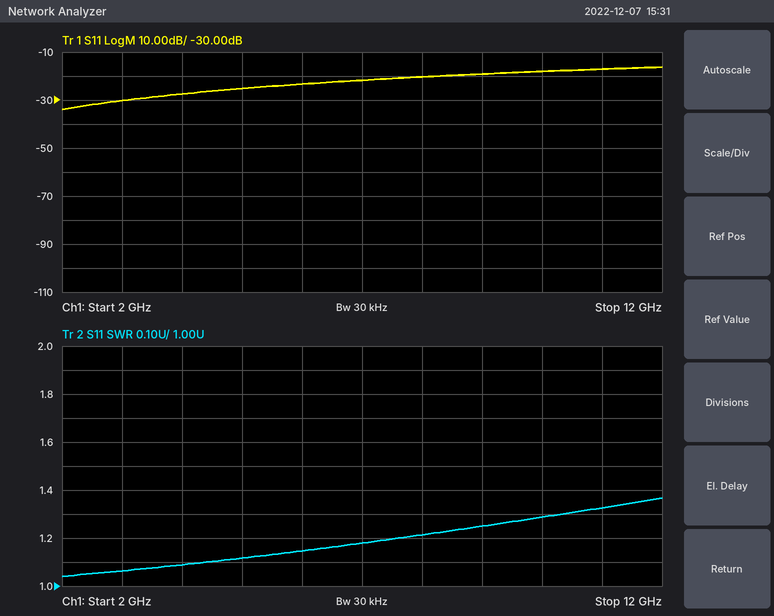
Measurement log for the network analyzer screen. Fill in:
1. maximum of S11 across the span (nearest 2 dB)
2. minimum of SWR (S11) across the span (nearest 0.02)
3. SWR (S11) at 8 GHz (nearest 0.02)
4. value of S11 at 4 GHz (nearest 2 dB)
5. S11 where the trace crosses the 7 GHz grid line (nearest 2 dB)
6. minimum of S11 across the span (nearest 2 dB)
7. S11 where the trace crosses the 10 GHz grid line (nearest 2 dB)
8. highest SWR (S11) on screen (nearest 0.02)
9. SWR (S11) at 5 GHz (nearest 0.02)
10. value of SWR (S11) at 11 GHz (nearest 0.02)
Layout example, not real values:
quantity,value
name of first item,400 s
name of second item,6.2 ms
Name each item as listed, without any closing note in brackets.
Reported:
quantity,value
maximum of S11 across the span,-16 dB
minimum of SWR (S11) across the span,1.04
SWR (S11) at 8 GHz,1.22
value of S11 at 4 GHz,-28 dB
S11 where the trace crosses the 7 GHz grid line,-22 dB
minimum of S11 across the span,-34 dB
S11 where the trace crosses the 10 GHz grid line,-18 dB
highest SWR (S11) on screen,1.36
SWR (S11) at 5 GHz,1.12
value of SWR (S11) at 11 GHz,1.32
